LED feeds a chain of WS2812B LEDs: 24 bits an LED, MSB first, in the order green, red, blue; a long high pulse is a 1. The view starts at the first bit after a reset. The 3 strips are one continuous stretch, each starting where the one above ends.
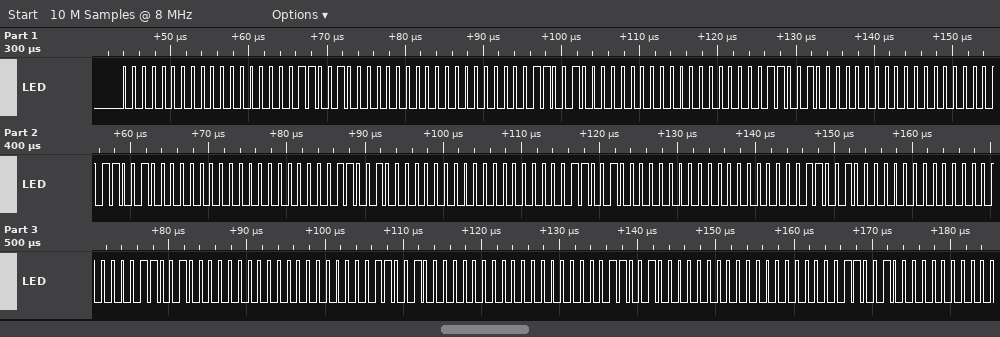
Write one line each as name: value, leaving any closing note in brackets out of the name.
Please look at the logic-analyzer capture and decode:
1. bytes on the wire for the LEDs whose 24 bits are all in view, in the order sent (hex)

bytes on the wire for the LEDs whose 24 bits are all in view, in the order sent: 00 00 32 00 00 32 00 00 32 00 00 32 00 00 32 00 00 32 00 00 32 00 00 32 00 00 32 00 00 32 00 00 32
